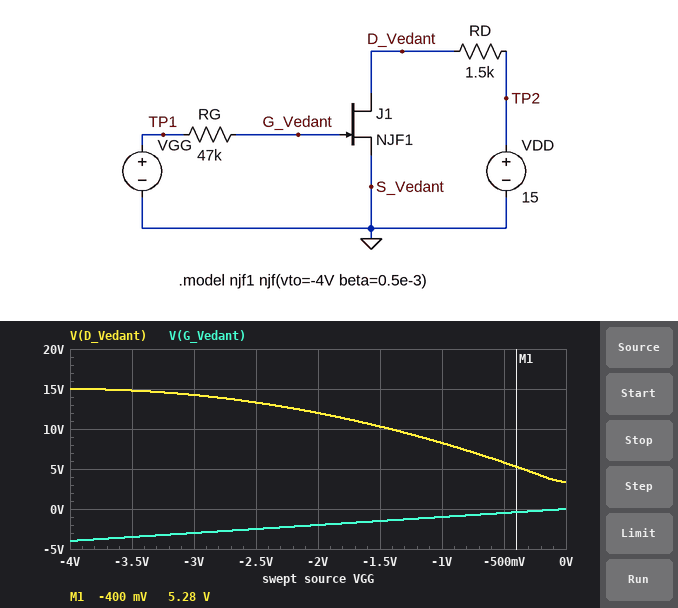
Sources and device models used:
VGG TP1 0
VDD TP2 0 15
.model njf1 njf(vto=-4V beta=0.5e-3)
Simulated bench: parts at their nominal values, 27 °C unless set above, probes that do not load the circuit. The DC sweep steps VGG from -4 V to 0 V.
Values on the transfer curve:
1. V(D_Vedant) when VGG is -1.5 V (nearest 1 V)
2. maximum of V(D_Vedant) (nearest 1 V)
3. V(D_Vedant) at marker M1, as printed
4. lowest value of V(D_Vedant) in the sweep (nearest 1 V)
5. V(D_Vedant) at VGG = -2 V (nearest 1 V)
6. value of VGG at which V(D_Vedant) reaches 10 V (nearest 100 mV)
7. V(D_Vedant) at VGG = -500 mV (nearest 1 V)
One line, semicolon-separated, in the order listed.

10 V; 15 V; 5.28 V; 3 V; 12 V; -1.4 V; 6 V
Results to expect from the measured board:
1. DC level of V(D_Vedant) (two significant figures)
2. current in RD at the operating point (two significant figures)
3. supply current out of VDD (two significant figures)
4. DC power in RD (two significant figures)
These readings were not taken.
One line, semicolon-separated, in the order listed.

3.3 V; 7.8 mA; 7.8 mA; 91 mW
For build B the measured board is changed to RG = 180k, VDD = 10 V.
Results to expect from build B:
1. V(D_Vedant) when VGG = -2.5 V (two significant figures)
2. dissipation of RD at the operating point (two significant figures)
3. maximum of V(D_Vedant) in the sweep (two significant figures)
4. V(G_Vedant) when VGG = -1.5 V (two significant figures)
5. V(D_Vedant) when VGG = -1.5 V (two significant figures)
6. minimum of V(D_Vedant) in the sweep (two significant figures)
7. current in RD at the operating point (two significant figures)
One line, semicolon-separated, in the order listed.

8.3 V; 45 mW; 10 V; -1.5 V; 5.3 V; 1.8 V; 5.5 mA
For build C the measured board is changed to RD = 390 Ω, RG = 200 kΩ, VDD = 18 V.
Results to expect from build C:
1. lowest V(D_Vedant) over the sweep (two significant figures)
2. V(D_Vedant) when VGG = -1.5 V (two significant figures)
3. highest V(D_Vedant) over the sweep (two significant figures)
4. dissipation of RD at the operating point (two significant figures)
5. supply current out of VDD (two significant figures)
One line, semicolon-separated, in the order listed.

15 V; 17 V; 18 V; 25 mW; 8.0 mA
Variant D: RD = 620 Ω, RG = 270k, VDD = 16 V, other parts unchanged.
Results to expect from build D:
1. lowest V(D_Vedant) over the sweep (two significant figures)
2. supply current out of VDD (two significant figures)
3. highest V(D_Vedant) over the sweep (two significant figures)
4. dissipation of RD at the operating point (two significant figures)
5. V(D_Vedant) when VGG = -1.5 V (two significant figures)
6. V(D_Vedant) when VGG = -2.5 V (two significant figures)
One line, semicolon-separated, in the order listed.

11 V; 8.0 mA; 16 V; 40 mW; 14 V; 15 V
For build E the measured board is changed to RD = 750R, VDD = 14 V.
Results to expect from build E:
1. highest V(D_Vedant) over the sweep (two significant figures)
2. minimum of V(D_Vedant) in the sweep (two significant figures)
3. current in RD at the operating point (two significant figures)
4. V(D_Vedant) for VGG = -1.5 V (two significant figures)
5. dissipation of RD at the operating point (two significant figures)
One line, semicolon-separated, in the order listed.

14 V; 8.0 V; 8.0 mA; 12 V; 48 mW
